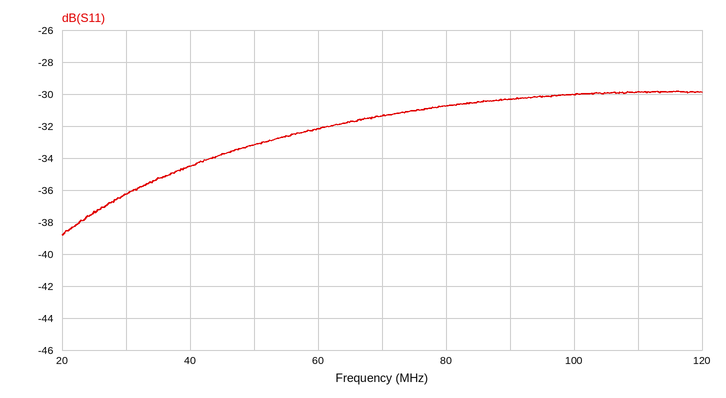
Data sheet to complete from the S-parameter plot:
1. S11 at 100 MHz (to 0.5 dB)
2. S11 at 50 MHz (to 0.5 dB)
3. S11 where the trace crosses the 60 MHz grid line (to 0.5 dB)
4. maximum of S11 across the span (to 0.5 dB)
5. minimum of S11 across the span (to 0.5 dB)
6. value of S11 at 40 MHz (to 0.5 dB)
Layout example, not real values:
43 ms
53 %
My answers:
-30.0 dB
-33.0 dB
-32.0 dB
-30.0 dB
-39.0 dB
-34.5 dB
